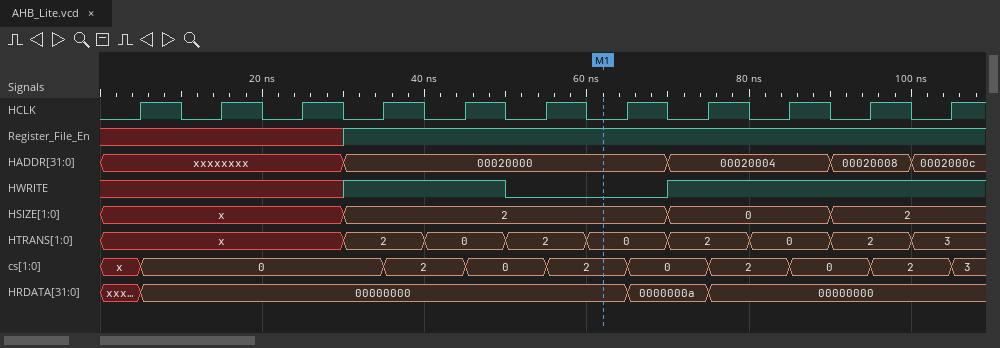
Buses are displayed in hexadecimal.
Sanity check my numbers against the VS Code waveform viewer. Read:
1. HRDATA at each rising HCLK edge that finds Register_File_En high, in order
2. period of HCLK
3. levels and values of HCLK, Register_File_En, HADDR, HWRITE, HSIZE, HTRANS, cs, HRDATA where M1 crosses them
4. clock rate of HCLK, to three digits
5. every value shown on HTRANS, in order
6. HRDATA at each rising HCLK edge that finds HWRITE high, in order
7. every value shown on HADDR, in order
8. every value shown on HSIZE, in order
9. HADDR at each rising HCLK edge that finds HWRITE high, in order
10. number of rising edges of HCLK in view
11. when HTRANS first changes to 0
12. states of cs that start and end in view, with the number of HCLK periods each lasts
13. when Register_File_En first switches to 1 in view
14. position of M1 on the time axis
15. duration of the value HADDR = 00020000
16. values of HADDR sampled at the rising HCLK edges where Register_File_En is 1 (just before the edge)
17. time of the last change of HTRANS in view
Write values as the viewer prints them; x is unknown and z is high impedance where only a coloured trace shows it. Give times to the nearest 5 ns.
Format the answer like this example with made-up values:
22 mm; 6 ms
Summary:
00000000, 00000000, 00000000, 00000000, 0000000a, 00000000, 00000000, 00000000; 10 ns; HCLK=0, Register_File_En=1, HADDR=00020000, HWRITE=0, HSIZE=2, HTRANS=0, cs=2, HRDATA=00000000; 100 MHz; x, 2, 0, 2, 0, 2, 0, 2, 3; 00000000, 00000000, 0000000a, 00000000, 00000000, 00000000; xxxxxxxx, 00020000, 00020004, 00020008, 0002000c; x, 2, 0, 2; 00020000, 00020000, 00020004, 00020004, 00020008, 0002000c; 11; 40 ns; 0: 3, 2: 1, 0: 1, 2: 1, 0: 1, 2: 1, 0: 1, 2: 1; 30 ns; 60 ns; 40 ns; 00020000, 00020000, 00020000, 00020000, 00020004, 00020004, 00020008, 0002000c; 100 ns
